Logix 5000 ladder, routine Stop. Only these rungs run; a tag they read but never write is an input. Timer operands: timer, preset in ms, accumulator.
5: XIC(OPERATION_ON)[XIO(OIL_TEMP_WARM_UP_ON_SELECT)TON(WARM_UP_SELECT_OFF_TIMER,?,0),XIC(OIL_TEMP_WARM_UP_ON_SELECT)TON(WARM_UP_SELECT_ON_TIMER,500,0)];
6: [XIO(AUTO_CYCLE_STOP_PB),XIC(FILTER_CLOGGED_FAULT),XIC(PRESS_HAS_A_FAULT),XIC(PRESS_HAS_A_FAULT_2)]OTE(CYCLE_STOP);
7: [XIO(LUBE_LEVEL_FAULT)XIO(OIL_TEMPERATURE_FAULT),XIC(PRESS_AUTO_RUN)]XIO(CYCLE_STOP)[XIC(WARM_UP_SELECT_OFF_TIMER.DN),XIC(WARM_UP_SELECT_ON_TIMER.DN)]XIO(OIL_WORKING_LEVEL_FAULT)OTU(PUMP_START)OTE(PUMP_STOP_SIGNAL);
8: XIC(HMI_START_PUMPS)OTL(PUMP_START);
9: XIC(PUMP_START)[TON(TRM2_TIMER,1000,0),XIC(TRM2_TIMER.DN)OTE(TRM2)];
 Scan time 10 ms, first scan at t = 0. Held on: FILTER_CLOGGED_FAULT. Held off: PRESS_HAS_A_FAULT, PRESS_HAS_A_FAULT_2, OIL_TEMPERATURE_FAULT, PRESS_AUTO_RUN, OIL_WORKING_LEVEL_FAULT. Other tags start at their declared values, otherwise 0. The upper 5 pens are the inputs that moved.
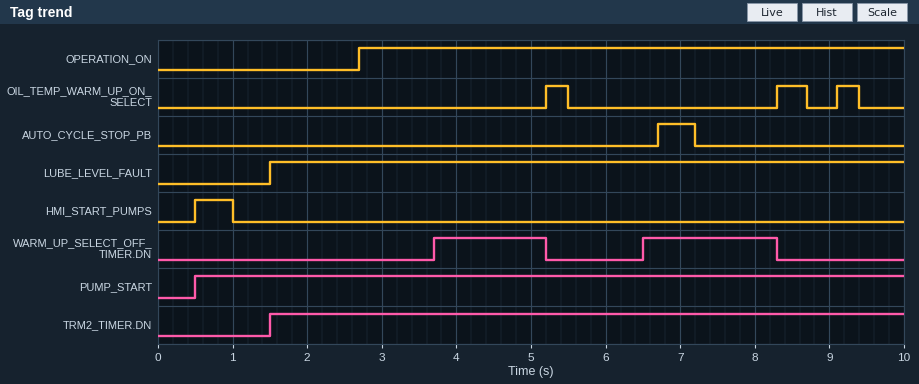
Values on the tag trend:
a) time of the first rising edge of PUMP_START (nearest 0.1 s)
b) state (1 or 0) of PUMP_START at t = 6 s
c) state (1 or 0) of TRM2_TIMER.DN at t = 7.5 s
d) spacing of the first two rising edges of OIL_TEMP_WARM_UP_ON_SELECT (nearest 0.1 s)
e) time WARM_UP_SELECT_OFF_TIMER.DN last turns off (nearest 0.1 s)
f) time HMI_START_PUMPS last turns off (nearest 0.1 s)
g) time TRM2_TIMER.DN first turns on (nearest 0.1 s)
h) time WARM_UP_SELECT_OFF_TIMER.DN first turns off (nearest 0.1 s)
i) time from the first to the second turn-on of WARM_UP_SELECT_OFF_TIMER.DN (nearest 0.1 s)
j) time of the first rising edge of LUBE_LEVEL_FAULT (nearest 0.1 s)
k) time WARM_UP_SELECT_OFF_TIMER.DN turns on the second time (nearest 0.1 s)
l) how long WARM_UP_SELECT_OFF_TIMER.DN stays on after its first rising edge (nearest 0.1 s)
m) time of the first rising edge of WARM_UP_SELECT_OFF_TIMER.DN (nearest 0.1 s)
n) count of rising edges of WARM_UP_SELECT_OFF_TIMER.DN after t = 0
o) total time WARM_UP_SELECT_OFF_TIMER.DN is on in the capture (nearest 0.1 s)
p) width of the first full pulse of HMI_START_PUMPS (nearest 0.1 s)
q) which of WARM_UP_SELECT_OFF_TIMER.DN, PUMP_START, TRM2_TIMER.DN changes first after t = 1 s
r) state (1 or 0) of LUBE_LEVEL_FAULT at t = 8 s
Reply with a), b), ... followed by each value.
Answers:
a) 0.5 s
b) 1
c) 1
d) 3.1 s
e) 8.3 s
f) 1.0 s
g) 1.5 s
h) 5.2 s
i) 2.8 s
j) 1.5 s
k) 6.5 s
l) 1.5 s
m) 3.7 s
n) 2
o) 3.3 s
p) 0.5 s
q) TRM2_TIMER.DN
r) 1
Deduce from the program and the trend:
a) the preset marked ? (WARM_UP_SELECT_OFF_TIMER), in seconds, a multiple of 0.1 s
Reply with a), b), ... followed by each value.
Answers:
a) 1.0 s
